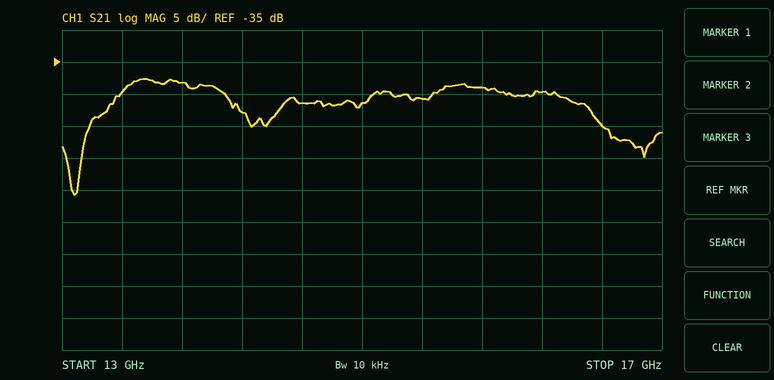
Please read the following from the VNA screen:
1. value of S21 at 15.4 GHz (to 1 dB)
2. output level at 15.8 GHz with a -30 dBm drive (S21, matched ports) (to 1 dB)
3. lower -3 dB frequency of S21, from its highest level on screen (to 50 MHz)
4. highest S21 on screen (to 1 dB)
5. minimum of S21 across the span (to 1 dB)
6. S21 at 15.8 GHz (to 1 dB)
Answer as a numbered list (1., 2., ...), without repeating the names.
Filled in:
1. -41 dB
2. -69 dBm
3. 13.35 GHz
4. -38 dB
5. -56 dB
6. -39 dB
